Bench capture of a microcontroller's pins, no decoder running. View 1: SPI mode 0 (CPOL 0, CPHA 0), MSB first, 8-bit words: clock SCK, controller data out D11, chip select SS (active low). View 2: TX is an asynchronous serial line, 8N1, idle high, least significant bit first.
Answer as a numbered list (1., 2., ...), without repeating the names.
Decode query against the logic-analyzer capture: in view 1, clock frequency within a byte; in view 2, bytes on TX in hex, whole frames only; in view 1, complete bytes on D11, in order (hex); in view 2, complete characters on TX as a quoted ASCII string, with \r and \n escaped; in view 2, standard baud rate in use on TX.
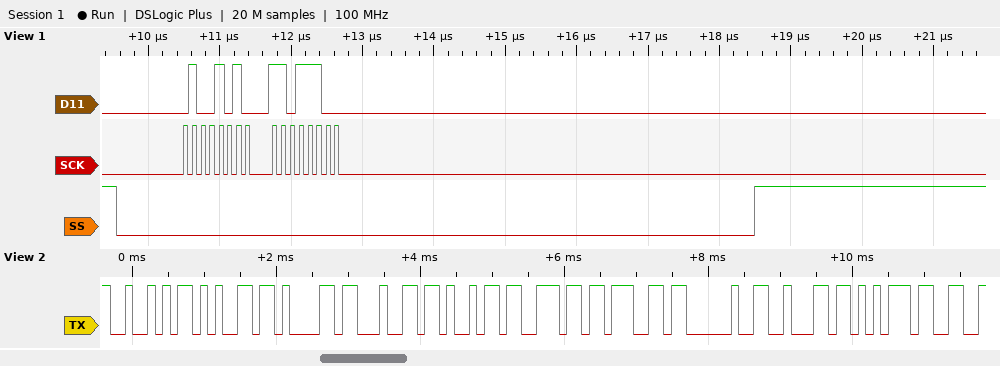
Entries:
1. 8 MHz
2. 52 65 61 64 69 6E 67 20 62 75
3. 4A DC
4. "Reading bu"
5. 9600 baud
